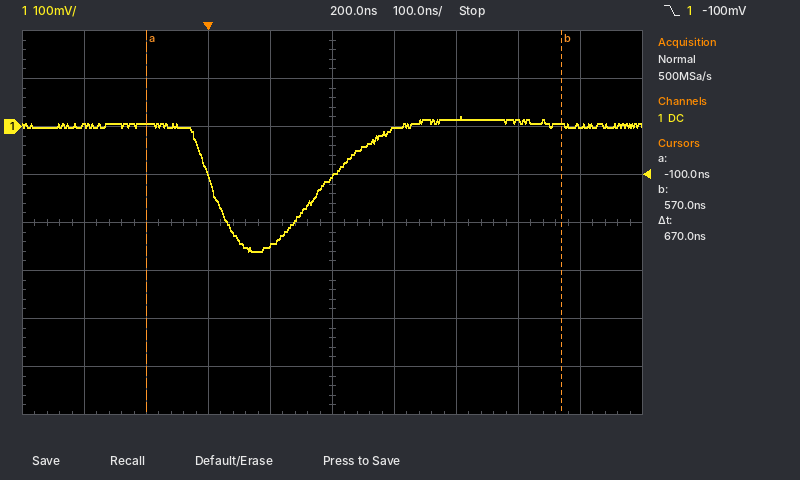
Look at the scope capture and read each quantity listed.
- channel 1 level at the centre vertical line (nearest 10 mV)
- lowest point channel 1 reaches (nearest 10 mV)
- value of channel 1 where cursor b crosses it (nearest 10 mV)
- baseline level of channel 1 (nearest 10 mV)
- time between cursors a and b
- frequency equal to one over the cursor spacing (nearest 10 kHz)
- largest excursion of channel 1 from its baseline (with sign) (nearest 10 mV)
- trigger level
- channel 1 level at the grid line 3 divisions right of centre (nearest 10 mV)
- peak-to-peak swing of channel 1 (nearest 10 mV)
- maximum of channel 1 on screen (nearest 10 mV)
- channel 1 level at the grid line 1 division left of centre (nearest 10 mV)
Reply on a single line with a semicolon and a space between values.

-110 mV; -260 mV; 0 mV; 0 mV; 670 ns; 1.49 MHz; -260 mV; -100 mV; 10 mV; 280 mV; 20 mV; -250 mV
